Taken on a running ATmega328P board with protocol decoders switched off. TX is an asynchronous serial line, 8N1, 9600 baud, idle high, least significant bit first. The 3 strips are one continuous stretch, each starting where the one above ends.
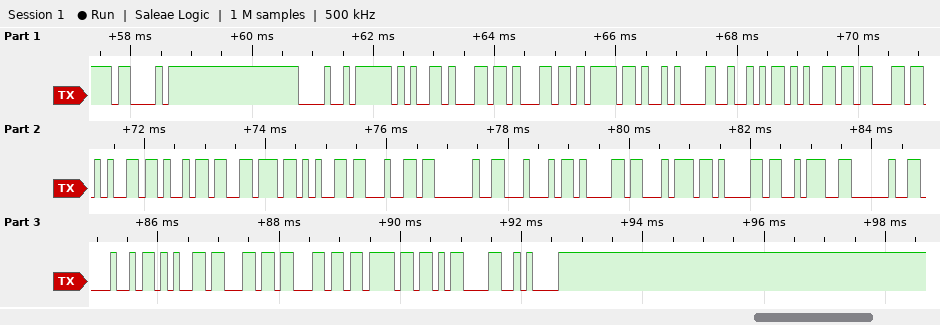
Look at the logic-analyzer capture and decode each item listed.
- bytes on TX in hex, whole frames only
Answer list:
43 48 65 6C 6C 6F 0A 52 65 63 65 69 76 65 64 20 44 61 74 61 3A 20 48 65 6C 6C 6F 0D 0A
